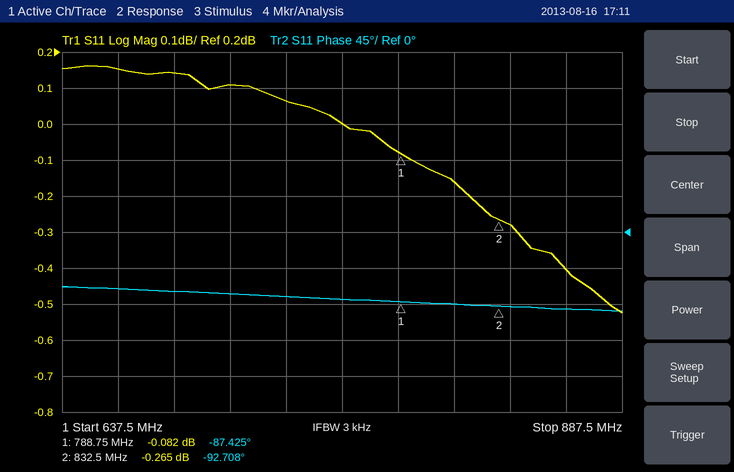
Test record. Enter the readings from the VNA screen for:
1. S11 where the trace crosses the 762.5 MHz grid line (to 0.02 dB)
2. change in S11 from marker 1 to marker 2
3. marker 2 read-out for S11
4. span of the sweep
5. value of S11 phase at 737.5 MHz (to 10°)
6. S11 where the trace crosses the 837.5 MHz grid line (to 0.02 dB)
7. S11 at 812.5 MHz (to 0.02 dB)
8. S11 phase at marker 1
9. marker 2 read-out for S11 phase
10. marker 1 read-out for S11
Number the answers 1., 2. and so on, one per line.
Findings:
1. 0.00 dB
2. -0.183 dB
3. -0.265 dB
4. 250 MHz
5. -80°
6. -0.28 dB
7. -0.16 dB
8. -87.425°
9. -92.708°
10. -0.082 dB
